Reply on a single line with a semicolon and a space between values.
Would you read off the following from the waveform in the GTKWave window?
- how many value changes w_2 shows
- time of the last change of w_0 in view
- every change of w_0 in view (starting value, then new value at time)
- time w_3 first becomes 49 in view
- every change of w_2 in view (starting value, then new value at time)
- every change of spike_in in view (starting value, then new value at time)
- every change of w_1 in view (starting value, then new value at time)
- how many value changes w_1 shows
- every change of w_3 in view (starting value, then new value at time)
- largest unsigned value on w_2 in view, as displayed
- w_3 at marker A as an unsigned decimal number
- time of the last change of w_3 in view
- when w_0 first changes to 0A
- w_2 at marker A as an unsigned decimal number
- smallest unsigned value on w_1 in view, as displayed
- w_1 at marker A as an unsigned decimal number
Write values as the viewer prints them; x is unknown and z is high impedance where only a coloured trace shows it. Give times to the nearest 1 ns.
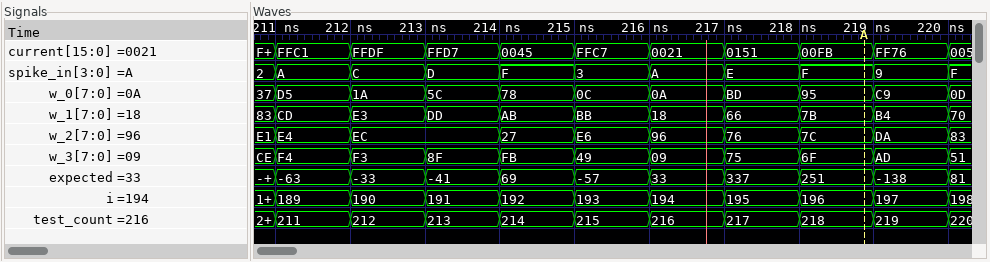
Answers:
9; 220 ns; 37, D5 at 211 ns, 1A at 212 ns, 5C at 213 ns, 78 at 214 ns, 0C at 215 ns, 0A at 216 ns, BD at 217 ns, 95 at 218 ns, C9 at 219 ns, 0D at 220 ns; 215 ns; E1, E4 at 211 ns, EC at 212 ns, 27 at 214 ns, E6 at 215 ns, 96 at 216 ns, 76 at 217 ns, 7C at 218 ns, DA at 219 ns, 83 at 220 ns; 2, A at 211 ns, C at 212 ns, D at 213 ns, F at 214 ns, 3 at 215 ns, A at 216 ns, E at 217 ns, F at 218 ns, 9 at 219 ns, F at 220 ns; 83, CD at 211 ns, E3 at 212 ns, DD at 213 ns, AB at 214 ns, BB at 215 ns, 18 at 216 ns, 66 at 217 ns, 7B at 218 ns, B4 at 219 ns, 70 at 220 ns; 10; CE, F4 at 211 ns, F3 at 212 ns, 8F at 213 ns, FB at 214 ns, 49 at 215 ns, 09 at 216 ns, 75 at 217 ns, 6F at 218 ns, AD at 219 ns, 51 at 220 ns; EC; 111; 220 ns; 216 ns; 124; 18; 123
